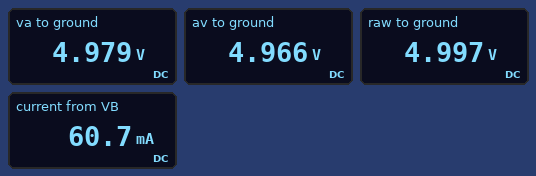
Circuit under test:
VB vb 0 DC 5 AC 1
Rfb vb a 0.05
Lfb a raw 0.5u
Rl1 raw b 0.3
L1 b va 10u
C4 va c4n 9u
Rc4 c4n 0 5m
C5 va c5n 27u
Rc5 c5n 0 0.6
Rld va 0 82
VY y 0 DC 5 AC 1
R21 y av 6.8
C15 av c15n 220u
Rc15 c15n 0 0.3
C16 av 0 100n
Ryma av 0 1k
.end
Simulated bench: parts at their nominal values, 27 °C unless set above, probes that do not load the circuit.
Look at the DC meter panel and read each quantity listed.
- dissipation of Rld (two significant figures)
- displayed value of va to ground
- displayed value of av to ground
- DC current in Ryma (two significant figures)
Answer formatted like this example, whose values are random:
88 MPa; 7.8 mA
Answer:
300 mW; 4.979 V; 4.966 V; 5.0 mA
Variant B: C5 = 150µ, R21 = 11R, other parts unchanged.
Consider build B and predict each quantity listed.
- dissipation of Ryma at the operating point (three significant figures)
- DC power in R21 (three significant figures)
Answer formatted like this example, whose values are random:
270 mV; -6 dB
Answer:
24.5 mW; 269 µW
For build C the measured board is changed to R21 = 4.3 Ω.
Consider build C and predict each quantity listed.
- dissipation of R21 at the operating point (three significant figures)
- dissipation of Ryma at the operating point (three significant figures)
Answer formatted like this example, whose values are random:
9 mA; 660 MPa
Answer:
107 µW; 24.8 mW
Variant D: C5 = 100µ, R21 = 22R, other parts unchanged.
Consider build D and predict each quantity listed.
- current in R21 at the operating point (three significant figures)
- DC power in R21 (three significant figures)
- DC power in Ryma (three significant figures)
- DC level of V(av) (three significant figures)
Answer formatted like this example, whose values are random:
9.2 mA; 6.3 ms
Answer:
4.89 mA; 527 µW; 23.9 mW; 4.89 V
